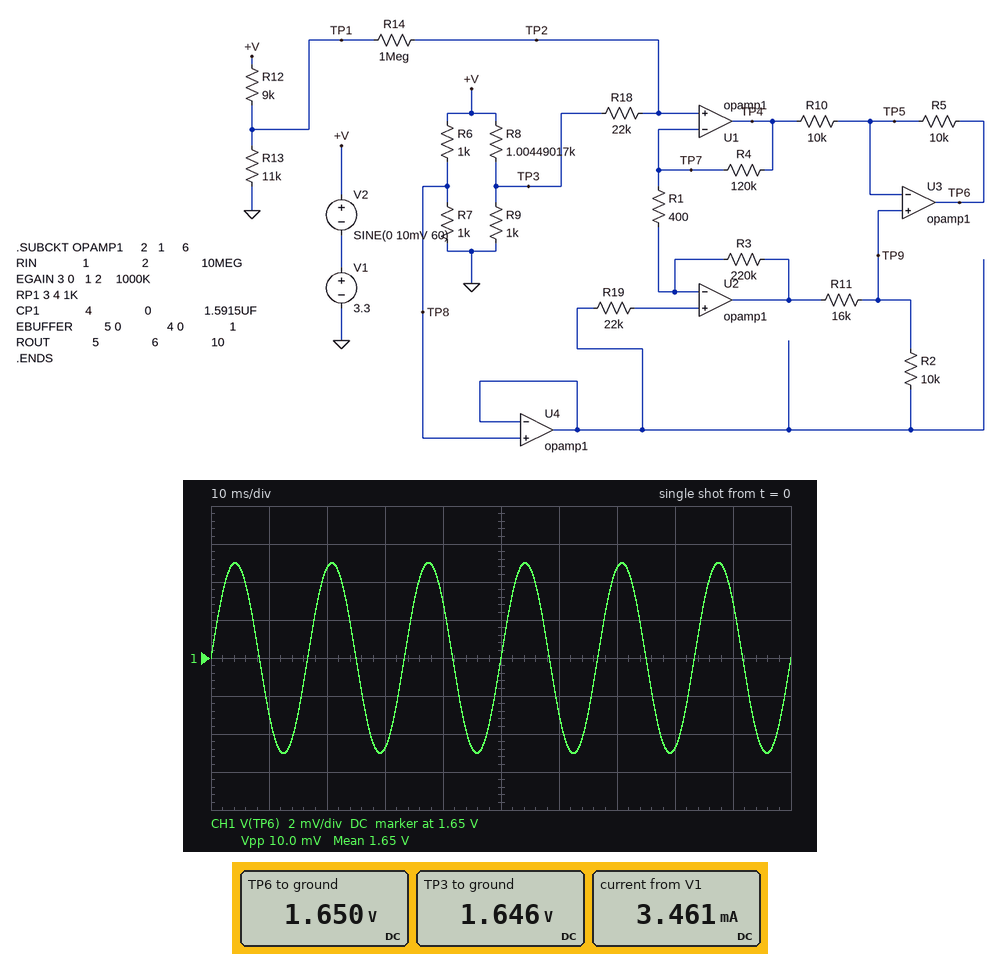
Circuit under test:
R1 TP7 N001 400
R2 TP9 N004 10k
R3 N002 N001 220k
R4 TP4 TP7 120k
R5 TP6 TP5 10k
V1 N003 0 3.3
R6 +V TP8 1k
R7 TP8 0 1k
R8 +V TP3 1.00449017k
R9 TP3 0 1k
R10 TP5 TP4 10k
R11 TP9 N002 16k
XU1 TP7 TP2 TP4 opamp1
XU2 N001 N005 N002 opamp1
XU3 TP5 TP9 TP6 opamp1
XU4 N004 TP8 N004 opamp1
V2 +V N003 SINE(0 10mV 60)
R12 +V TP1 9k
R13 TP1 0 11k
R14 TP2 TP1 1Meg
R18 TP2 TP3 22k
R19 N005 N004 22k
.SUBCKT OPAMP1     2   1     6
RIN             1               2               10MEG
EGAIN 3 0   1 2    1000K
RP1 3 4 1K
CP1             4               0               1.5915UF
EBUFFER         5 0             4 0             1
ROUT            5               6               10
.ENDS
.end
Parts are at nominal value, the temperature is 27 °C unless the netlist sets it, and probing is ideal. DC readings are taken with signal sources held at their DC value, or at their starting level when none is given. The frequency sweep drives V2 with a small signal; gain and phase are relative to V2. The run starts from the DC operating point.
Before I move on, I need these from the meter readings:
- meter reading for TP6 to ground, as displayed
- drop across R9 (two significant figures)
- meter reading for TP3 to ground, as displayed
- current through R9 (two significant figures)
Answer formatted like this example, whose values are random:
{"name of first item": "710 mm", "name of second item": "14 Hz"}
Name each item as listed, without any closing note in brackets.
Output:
{"meter reading for TP6 to ground, as displayed": "1.650 V", "drop across R9": "1.6 V", "meter reading for TP3 to ground, as displayed": "1.646 V", "current through R9": "1.6 mA"}
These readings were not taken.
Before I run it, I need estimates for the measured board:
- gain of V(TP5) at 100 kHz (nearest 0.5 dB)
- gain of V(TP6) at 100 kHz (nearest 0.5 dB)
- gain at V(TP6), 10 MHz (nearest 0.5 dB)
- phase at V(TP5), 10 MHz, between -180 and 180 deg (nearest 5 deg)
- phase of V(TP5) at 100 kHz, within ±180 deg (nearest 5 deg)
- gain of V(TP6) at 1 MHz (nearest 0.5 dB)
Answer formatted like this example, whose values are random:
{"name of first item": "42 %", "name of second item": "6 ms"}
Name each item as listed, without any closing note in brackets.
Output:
{"gain of V(TP5) at 100 kHz": "-7.0 dB", "gain of V(TP6) at 100 kHz": "-8.5 dB", "gain at V(TP6), 10 MHz": "-22.5 dB", "phase at V(TP5), 10 MHz, between -180 and 180 deg": "-10 deg", "phase of V(TP5) at 100 kHz, within ±180 deg": "-10 deg", "gain of V(TP6) at 1 MHz": "-20.5 dB"}
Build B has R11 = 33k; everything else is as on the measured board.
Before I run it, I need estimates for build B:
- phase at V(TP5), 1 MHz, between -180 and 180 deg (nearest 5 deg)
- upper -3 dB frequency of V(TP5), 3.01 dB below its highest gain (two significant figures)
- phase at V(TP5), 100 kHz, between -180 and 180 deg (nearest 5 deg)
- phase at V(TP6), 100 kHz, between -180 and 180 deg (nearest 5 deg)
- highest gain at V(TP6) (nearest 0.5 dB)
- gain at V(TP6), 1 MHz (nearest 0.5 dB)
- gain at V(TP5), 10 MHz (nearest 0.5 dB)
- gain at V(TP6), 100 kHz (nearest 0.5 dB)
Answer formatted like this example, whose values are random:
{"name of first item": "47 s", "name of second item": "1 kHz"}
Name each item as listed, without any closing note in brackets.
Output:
{"phase at V(TP5), 1 MHz, between -180 and 180 deg": "0 deg", "upper -3 dB frequency of V(TP5), 3.01 dB below its highest gain": "46 MHz", "phase at V(TP5), 100 kHz, between -180 and 180 deg": "-5 deg", "phase at V(TP6), 100 kHz, between -180 and 180 deg": "-25 deg", "highest gain at V(TP6)": "-6.0 dB", "gain at V(TP6), 1 MHz": "-15.0 dB", "gain at V(TP5), 10 MHz": "-7.5 dB", "gain at V(TP6), 100 kHz": "-8.0 dB"}
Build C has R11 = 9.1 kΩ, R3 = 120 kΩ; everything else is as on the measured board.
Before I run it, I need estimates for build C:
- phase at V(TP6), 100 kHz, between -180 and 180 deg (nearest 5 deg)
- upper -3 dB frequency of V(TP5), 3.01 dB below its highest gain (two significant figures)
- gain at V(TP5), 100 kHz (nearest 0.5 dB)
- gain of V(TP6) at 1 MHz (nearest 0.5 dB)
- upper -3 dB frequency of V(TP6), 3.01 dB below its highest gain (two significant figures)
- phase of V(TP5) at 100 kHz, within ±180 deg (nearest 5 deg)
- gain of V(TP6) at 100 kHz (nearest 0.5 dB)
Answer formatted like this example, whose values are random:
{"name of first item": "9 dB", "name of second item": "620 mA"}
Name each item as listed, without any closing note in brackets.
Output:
{"phase at V(TP6), 100 kHz, between -180 and 180 deg": "-30 deg", "upper -3 dB frequency of V(TP5), 3.01 dB below its highest gain": "24 MHz", "gain at V(TP5), 100 kHz": "-6.5 dB", "gain of V(TP6) at 1 MHz": "-21.5 dB", "upper -3 dB frequency of V(TP6), 3.01 dB below its highest gain": "170 kHz", "phase of V(TP5) at 100 kHz, within ±180 deg": "-5 deg", "gain of V(TP6) at 100 kHz": "-7.5 dB"}
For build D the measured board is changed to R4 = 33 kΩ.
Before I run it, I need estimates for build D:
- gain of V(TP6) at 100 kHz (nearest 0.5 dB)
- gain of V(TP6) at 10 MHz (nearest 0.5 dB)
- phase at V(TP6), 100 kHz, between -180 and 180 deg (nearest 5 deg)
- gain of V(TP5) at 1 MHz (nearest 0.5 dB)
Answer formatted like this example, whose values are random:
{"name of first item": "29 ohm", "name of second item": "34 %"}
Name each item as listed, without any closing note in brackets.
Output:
{"gain of V(TP6) at 100 kHz": "-7.5 dB", "gain of V(TP6) at 10 MHz": "-20.0 dB", "phase at V(TP6), 100 kHz, between -180 and 180 deg": "-25 deg", "gain of V(TP5) at 1 MHz": "-9.5 dB"}
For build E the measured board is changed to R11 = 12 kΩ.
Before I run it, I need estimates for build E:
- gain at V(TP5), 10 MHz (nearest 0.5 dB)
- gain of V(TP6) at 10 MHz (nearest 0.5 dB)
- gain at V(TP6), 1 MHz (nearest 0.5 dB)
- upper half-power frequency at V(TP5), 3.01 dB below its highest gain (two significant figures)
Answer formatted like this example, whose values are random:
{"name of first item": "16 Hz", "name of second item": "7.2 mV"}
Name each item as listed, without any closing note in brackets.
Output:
{"gain at V(TP5), 10 MHz": "-9.0 dB", "gain of V(TP6) at 10 MHz": "-30.5 dB", "gain at V(TP6), 1 MHz": "-23.5 dB", "upper half-power frequency at V(TP5), 3.01 dB below its highest gain": "1.8 MHz"}
